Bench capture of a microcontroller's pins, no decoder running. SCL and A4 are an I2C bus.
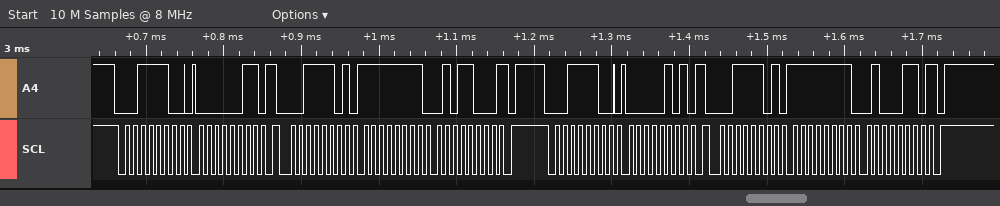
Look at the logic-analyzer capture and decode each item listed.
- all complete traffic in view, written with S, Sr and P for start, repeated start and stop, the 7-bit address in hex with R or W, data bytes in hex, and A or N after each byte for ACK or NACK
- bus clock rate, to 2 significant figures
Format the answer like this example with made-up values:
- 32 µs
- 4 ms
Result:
- S 1EW A 03 A Sr 1ER A FF A 58 N P S 1EW A 05 A Sr 1ER A FF A 46 N P
- 100 kHz
